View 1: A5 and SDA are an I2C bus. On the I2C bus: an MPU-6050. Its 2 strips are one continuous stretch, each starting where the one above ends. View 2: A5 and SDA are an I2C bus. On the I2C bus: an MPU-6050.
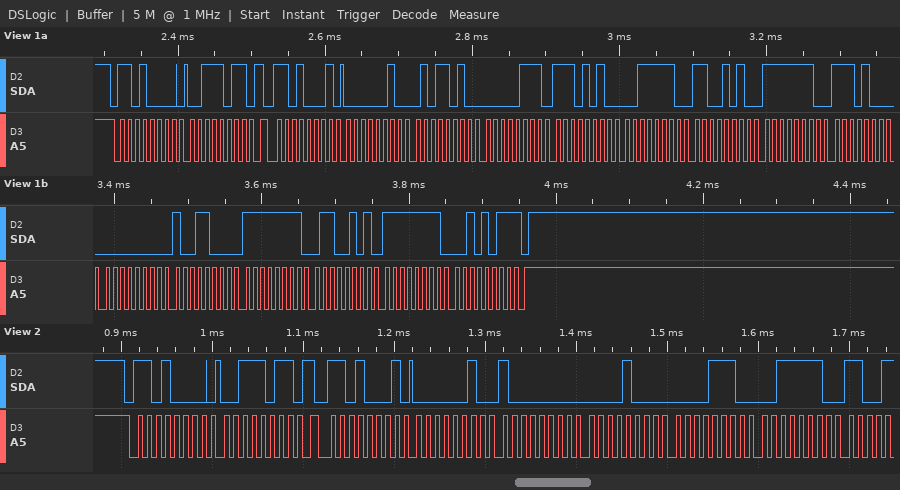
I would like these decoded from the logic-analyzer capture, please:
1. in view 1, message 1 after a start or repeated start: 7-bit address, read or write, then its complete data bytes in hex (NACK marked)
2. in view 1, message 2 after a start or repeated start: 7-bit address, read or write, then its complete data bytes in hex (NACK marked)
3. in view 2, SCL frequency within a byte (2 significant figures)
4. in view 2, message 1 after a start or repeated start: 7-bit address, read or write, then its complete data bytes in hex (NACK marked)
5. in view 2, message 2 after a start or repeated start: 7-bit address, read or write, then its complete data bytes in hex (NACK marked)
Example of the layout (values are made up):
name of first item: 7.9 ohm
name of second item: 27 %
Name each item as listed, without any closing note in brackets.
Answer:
in view 1, message 1 after a start or repeated start: 7-bit address, read or write, then its complete data bytes in hex: 0x68 write: 3B
in view 1, message 2 after a start or repeated start: 7-bit address, read or write, then its complete data bytes in hex: 0x68 read: 02 5A 07 EA 3E CA FE E8 00 98 FF 65 FF 2B NACK
in view 2, SCL frequency within a byte: 100 kHz
in view 2, message 1 after a start or repeated start: 7-bit address, read or write, then its complete data bytes in hex: 0x68 write: 3B
in view 2, message 2 after a start or repeated start: 7-bit address, read or write, then its complete data bytes in hex: 0x68 read: 02 80 08 0E 3E
